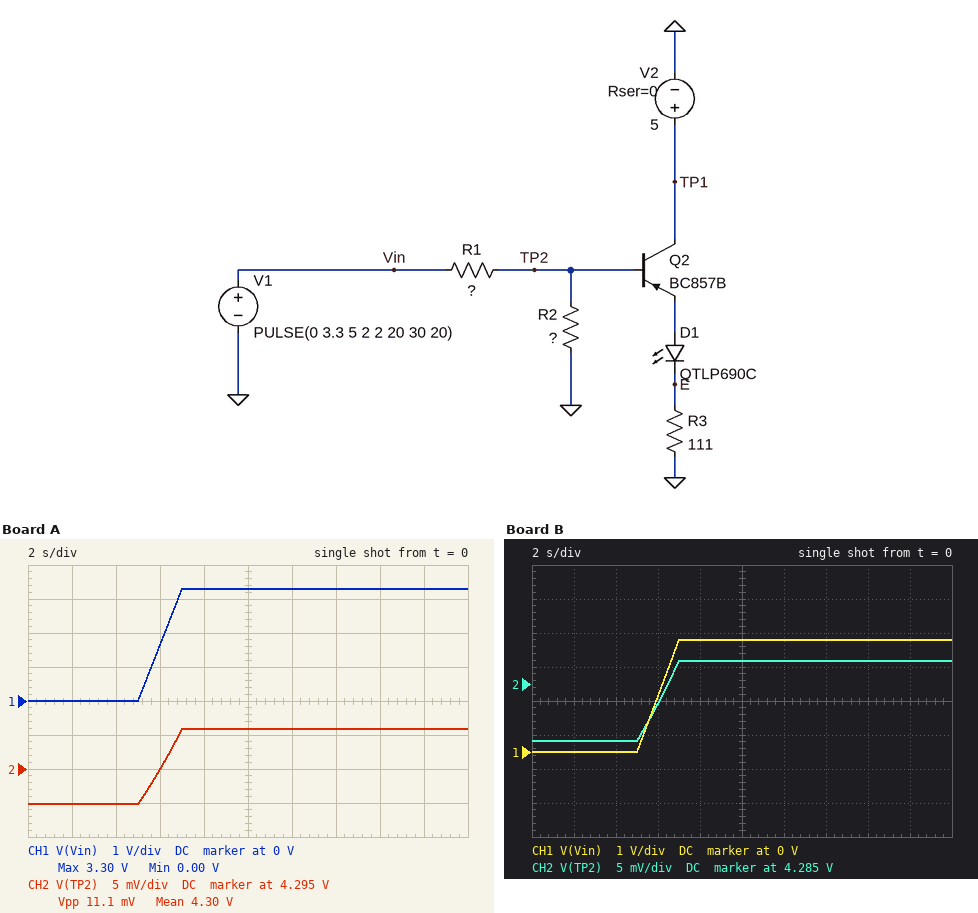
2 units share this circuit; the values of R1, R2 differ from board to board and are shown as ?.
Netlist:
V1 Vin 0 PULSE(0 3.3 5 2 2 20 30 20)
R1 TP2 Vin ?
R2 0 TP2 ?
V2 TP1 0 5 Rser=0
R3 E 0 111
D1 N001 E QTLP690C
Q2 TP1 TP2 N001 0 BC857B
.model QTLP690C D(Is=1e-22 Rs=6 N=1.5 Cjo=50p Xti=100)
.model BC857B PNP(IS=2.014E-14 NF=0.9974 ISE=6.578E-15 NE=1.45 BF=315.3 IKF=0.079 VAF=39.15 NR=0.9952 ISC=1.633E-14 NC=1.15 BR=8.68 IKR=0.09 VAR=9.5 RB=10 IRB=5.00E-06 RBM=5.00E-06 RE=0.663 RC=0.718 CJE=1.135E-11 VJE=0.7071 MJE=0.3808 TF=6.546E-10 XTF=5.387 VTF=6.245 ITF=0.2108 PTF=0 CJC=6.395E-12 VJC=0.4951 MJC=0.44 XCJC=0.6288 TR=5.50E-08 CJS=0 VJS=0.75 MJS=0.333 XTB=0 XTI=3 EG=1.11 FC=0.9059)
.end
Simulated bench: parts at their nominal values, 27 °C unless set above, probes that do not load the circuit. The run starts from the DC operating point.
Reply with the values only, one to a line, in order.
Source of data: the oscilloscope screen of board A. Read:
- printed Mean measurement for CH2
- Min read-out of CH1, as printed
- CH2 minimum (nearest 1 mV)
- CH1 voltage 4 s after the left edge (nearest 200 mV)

4.30 V
0.00 V
4.290 V
0 V
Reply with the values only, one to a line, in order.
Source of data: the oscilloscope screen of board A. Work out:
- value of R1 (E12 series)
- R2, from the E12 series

6.8 kΩ
3.9 kΩ
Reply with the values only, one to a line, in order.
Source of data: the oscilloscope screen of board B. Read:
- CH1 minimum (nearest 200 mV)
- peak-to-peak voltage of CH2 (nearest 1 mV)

0 V
12 mV
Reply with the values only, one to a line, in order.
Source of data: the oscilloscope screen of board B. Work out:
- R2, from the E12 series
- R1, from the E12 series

2.7 kΩ
4.7 kΩ
